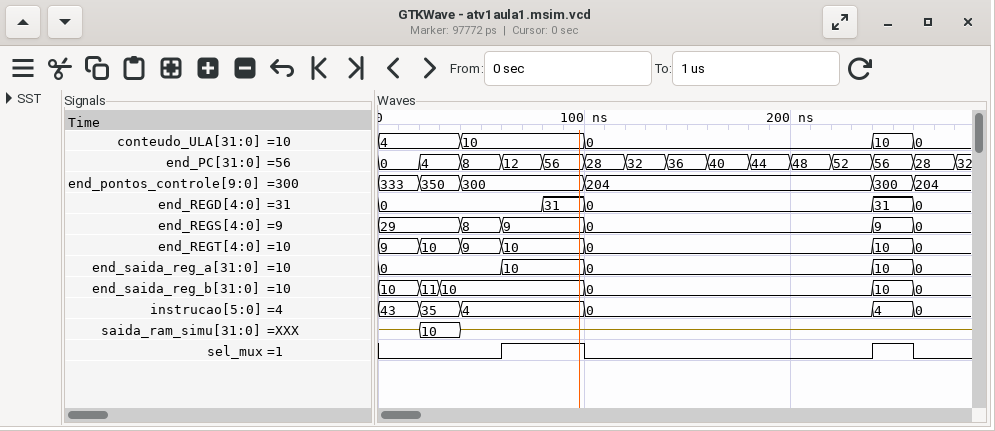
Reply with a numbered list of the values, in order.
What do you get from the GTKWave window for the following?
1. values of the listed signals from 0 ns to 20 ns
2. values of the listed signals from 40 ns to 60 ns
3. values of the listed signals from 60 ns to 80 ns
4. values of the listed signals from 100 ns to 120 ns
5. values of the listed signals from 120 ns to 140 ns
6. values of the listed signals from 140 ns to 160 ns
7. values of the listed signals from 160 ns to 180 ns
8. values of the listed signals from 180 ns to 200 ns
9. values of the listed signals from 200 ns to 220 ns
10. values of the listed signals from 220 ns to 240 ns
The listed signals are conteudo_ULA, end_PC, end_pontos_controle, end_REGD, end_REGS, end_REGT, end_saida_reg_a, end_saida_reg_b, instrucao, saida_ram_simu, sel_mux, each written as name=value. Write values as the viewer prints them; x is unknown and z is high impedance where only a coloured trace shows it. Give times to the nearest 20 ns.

1. conteudo_ULA=4, end_PC=0, end_pontos_controle=333, end_REGD=0, end_REGS=29, end_REGT=9, end_saida_reg_a=0, end_saida_reg_b=10, instrucao=43, saida_ram_simu=z, sel_mux=0
2. conteudo_ULA=10, end_PC=8, end_pontos_controle=300, end_REGD=0, end_REGS=8, end_REGT=9, end_saida_reg_a=0, end_saida_reg_b=10, instrucao=4, saida_ram_simu=z, sel_mux=0
3. conteudo_ULA=10, end_PC=12, end_pontos_controle=300, end_REGD=0, end_REGS=9, end_REGT=10, end_saida_reg_a=10, end_saida_reg_b=10, instrucao=4, saida_ram_simu=z, sel_mux=1
4. conteudo_ULA=0, end_PC=28, end_pontos_controle=204, end_REGD=0, end_REGS=0, end_REGT=0, end_saida_reg_a=0, end_saida_reg_b=0, instrucao=0, saida_ram_simu=z, sel_mux=0
5. conteudo_ULA=0, end_PC=32, end_pontos_controle=204, end_REGD=0, end_REGS=0, end_REGT=0, end_saida_reg_a=0, end_saida_reg_b=0, instrucao=0, saida_ram_simu=z, sel_mux=0
6. conteudo_ULA=0, end_PC=36, end_pontos_controle=204, end_REGD=0, end_REGS=0, end_REGT=0, end_saida_reg_a=0, end_saida_reg_b=0, instrucao=0, saida_ram_simu=z, sel_mux=0
7. conteudo_ULA=0, end_PC=40, end_pontos_controle=204, end_REGD=0, end_REGS=0, end_REGT=0, end_saida_reg_a=0, end_saida_reg_b=0, instrucao=0, saida_ram_simu=z, sel_mux=0
8. conteudo_ULA=0, end_PC=44, end_pontos_controle=204, end_REGD=0, end_REGS=0, end_REGT=0, end_saida_reg_a=0, end_saida_reg_b=0, instrucao=0, saida_ram_simu=z, sel_mux=0
9. conteudo_ULA=0, end_PC=48, end_pontos_controle=204, end_REGD=0, end_REGS=0, end_REGT=0, end_saida_reg_a=0, end_saida_reg_b=0, instrucao=0, saida_ram_simu=z, sel_mux=0
10. conteudo_ULA=0, end_PC=52, end_pontos_controle=204, end_REGD=0, end_REGS=0, end_REGT=0, end_saida_reg_a=0, end_saida_reg_b=0, instrucao=0, saida_ram_simu=z, sel_mux=0
